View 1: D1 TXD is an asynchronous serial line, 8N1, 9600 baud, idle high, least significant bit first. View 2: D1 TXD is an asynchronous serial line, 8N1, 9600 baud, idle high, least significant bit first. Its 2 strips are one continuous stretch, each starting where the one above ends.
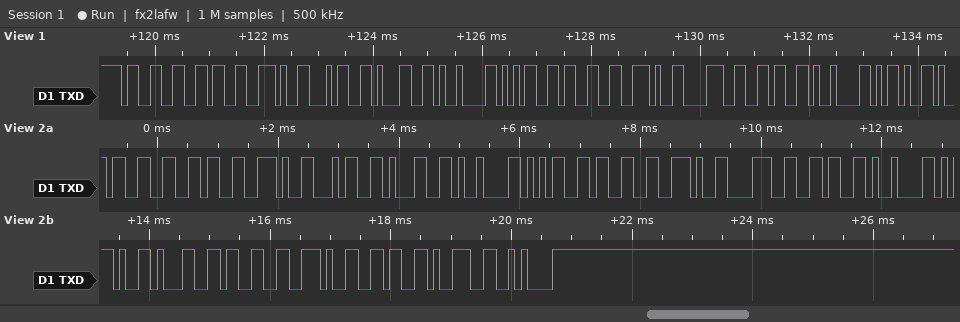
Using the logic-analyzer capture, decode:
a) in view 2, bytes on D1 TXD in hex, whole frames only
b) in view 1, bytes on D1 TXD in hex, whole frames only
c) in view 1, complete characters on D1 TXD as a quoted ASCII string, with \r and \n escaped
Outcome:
33 36 2E 34 31 09 35 33 2E 38 36 09 2D 31 33 2E 36 39 0A
33 36 2E 34 31 09 35 33 2E 38 36 09 2D
"36.41\t53.86\t-"
